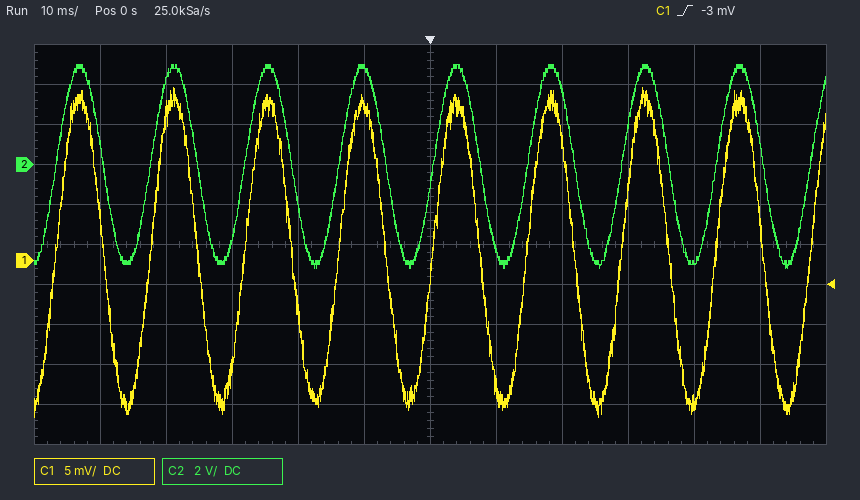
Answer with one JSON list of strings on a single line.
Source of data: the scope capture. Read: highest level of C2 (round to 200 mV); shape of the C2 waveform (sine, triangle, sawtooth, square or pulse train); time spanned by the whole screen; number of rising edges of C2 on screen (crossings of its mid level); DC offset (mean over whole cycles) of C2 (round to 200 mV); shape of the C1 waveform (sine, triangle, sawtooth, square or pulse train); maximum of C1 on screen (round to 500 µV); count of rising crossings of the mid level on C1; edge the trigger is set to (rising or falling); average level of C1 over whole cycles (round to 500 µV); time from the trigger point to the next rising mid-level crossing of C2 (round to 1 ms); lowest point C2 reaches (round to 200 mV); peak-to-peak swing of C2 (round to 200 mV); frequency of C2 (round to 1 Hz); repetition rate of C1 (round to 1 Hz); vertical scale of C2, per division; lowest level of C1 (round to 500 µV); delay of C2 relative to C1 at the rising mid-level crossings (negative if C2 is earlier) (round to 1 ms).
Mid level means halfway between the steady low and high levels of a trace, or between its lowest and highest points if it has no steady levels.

["5.0 V", "sine", "120 ms", "9", "0.0 V", "sine", "21.5 mV", "9", "rising", "1.0 mV", "15 ms", "-5.2 V", "10.2 V", "70 Hz", "70 Hz", "2 V", "-19.5 mV", "0 ms"]
